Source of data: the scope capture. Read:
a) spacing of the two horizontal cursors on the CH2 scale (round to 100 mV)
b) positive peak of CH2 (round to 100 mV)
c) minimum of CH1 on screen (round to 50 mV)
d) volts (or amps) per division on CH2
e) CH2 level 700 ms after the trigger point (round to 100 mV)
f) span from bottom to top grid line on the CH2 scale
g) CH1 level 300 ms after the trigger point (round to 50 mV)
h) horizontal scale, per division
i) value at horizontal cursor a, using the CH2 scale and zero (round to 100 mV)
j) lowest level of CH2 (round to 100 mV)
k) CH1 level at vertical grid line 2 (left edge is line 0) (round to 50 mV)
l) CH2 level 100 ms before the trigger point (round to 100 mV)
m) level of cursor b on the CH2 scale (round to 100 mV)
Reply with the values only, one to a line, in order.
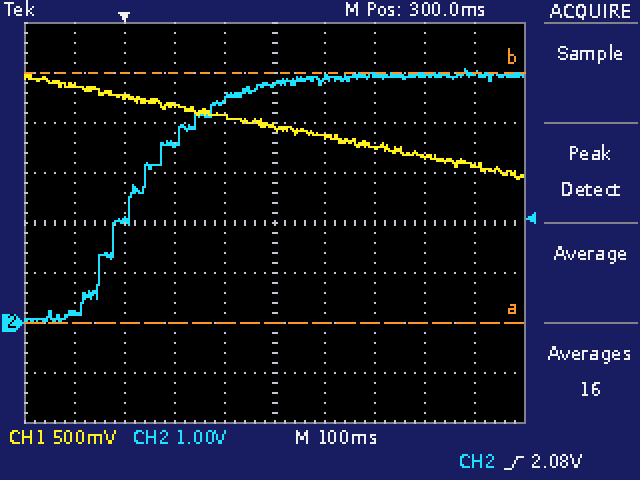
5.0 V
5.1 V
1.45 V
1 V
5.0 V
8 V
1.95 V
100 ms
0.0 V
0.0 V
2.25 V
200 mV
5.0 V
